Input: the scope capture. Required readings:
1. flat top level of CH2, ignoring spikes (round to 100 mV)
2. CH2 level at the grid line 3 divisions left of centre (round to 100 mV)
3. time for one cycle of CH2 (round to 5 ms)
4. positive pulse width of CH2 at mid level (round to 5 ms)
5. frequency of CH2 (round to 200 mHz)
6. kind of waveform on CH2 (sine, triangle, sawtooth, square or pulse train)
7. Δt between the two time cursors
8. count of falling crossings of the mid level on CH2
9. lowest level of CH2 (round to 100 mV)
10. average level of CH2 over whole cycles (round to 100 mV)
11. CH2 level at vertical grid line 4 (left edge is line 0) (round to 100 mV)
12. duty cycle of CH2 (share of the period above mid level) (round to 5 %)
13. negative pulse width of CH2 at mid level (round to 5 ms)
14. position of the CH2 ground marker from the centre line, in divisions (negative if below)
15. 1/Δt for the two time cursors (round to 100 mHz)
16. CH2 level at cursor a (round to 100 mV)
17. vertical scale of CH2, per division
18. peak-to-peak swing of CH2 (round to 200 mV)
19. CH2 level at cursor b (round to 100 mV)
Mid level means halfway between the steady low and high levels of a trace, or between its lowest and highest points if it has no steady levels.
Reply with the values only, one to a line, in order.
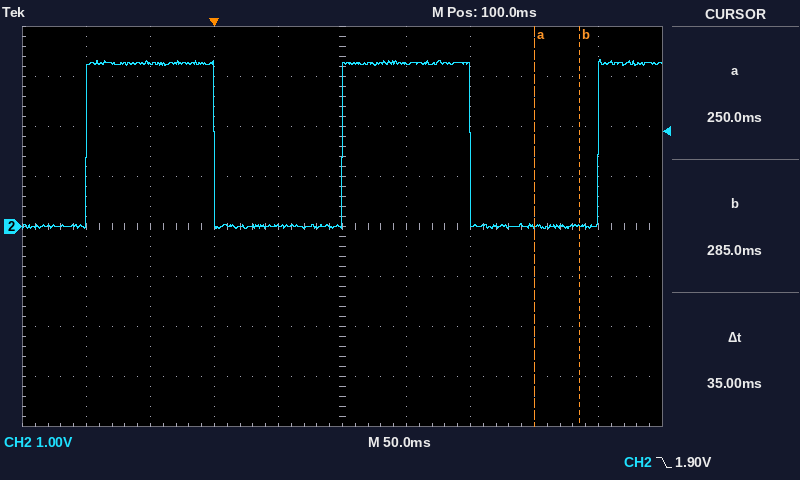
3.3 V
3.3 V
200 ms
100 ms
5.0 Hz
square
35 ms
2
0.0 V
1.6 V
0.0 V
50 %
100 ms
0.0 div
28.6 Hz
0.0 V
1 V
3.4 V
0.0 V
